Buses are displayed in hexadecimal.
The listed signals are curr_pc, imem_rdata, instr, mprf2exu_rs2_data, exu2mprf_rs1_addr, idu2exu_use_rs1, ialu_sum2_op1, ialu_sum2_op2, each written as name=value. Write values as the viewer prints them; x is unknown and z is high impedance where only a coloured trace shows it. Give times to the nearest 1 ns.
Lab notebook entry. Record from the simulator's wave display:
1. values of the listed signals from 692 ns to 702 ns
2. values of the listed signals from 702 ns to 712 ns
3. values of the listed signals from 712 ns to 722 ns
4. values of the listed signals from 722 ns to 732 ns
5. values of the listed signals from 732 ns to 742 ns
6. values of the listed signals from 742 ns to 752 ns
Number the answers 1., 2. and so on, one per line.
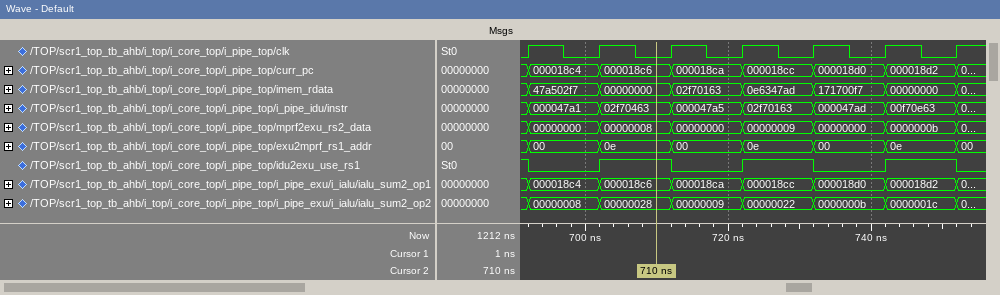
1. curr_pc=000018c4, imem_rdata=47a502f7, instr=000047a1, mprf2exu_rs2_data=00000000, exu2mprf_rs1_addr=00, idu2exu_use_rs1=0, ialu_sum2_op1=000018c4, ialu_sum2_op2=00000008
2. curr_pc=000018c6, imem_rdata=00000000, instr=02f70463, mprf2exu_rs2_data=00000008, exu2mprf_rs1_addr=0e, idu2exu_use_rs1=1, ialu_sum2_op1=000018c6, ialu_sum2_op2=00000028
3. curr_pc=000018ca, imem_rdata=02f70163, instr=000047a5, mprf2exu_rs2_data=00000000, exu2mprf_rs1_addr=00, idu2exu_use_rs1=0, ialu_sum2_op1=000018ca, ialu_sum2_op2=00000009
4. curr_pc=000018cc, imem_rdata=0e6347ad, instr=02f70163, mprf2exu_rs2_data=00000009, exu2mprf_rs1_addr=0e, idu2exu_use_rs1=1, ialu_sum2_op1=000018cc, ialu_sum2_op2=00000022
5. curr_pc=000018d0, imem_rdata=171700f7, instr=000047ad, mprf2exu_rs2_data=00000000, exu2mprf_rs1_addr=00, idu2exu_use_rs1=0, ialu_sum2_op1=000018d0, ialu_sum2_op2=0000000b
6. curr_pc=000018d2, imem_rdata=00000000, instr=00f70e63, mprf2exu_rs2_data=0000000b, exu2mprf_rs1_addr=0e, idu2exu_use_rs1=1, ialu_sum2_op1=000018d2, ialu_sum2_op2=0000001c
